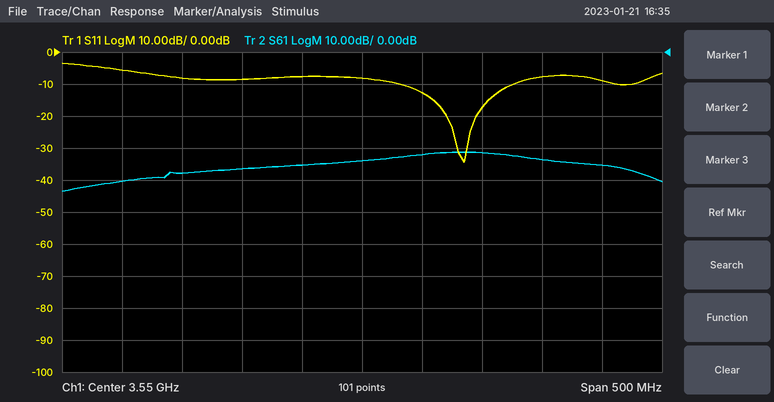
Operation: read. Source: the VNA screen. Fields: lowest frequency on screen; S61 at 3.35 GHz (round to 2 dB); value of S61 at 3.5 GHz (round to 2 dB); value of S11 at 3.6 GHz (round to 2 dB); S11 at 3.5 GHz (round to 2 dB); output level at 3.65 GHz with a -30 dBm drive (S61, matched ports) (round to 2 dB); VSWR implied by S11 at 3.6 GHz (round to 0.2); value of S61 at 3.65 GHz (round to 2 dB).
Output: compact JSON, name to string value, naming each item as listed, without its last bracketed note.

{"lowest frequency on screen": "3.3 GHz", "S61 at 3.35 GHz": "-40 dB", "value of S61 at 3.5 GHz": "-36 dB", "value of S11 at 3.6 GHz": "-12 dB", "S11 at 3.5 GHz": "-8 dB", "output level at 3.65 GHz with a -30 dBm drive (S61, matched ports)": "-62 dBm", "VSWR implied by S11 at 3.6 GHz": "1.6", "value of S61 at 3.65 GHz": "-32 dB"}
